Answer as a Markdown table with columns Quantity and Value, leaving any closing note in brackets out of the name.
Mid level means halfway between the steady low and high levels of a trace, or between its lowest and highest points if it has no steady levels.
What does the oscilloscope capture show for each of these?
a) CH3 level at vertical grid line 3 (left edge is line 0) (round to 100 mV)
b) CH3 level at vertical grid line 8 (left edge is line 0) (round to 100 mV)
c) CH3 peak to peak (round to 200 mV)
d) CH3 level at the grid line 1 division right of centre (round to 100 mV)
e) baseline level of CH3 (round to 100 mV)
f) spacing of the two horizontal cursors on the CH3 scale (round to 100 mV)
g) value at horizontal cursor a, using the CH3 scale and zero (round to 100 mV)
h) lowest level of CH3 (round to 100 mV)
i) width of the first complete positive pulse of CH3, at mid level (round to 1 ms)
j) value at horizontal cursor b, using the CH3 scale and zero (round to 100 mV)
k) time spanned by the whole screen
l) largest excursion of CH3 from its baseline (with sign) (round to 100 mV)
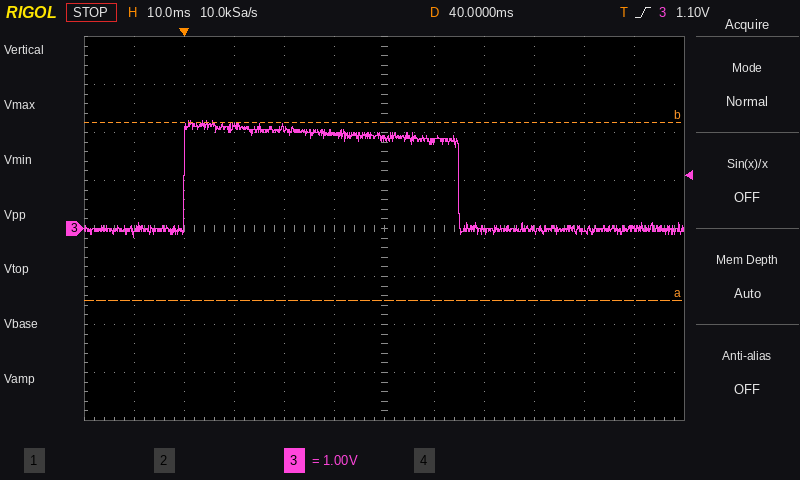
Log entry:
| Quantity | Value |
|---|---|
| CH3 level at vertical grid line 3 (left edge is line 0) | 2.1 V |
| CH3 level at vertical grid line 8 (left edge is line 0) | 0.0 V |
| CH3 peak to peak | 2.4 V |
| CH3 level at the grid line 1 division right of centre | 1.8 V |
| baseline level of CH3 | 0.0 V |
| spacing of the two horizontal cursors on the CH3 scale | 3.7 V |
| value at horizontal cursor a, using the CH3 scale and zero | -1.5 V |
| lowest level of CH3 | -200 mV |
| width of the first complete positive pulse of CH3, at mid level | 55 ms |
| value at horizontal cursor b, using the CH3 scale and zero | 2.2 V |
| time spanned by the whole screen | 120 ms |
| largest excursion of CH3 from its baseline (with sign) | +2.3 V |
